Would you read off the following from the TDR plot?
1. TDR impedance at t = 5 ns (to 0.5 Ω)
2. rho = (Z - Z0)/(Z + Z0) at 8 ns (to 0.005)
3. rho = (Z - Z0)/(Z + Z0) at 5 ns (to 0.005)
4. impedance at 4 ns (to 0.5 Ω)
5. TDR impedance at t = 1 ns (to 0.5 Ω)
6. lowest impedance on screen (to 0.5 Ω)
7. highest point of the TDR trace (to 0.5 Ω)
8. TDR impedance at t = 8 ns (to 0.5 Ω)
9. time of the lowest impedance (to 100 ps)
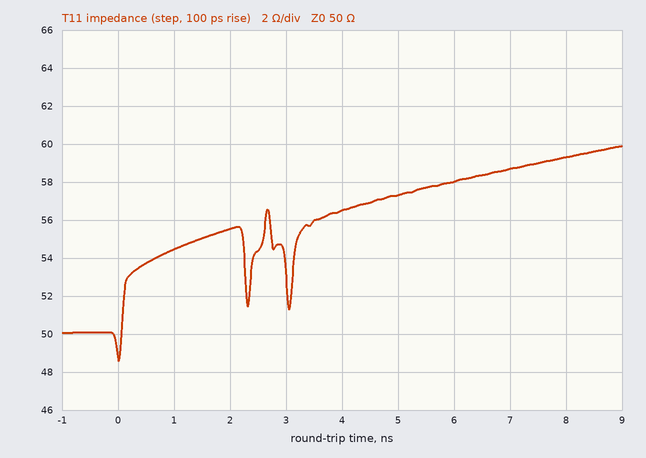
57.5 Ω
+0.085
+0.070
56.5 Ω
54.5 Ω
48.5 Ω
60.0 Ω
59.5 Ω
0.0 ns
